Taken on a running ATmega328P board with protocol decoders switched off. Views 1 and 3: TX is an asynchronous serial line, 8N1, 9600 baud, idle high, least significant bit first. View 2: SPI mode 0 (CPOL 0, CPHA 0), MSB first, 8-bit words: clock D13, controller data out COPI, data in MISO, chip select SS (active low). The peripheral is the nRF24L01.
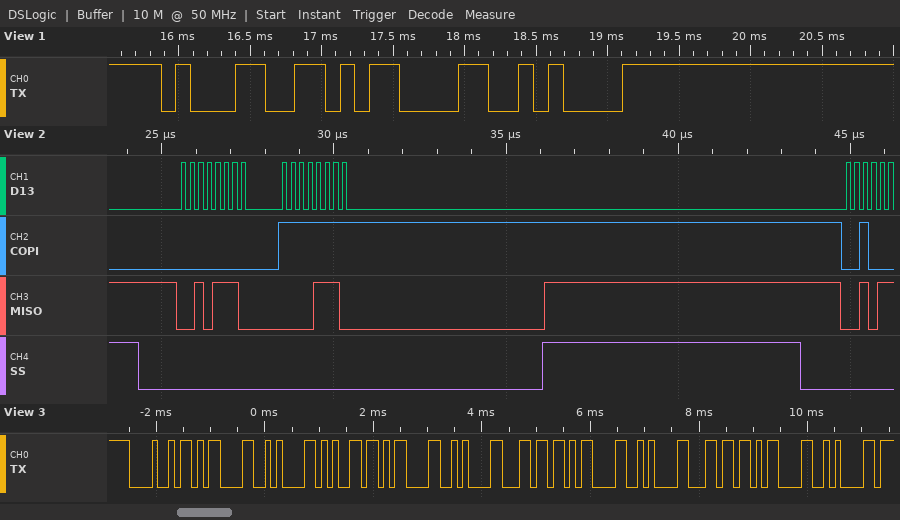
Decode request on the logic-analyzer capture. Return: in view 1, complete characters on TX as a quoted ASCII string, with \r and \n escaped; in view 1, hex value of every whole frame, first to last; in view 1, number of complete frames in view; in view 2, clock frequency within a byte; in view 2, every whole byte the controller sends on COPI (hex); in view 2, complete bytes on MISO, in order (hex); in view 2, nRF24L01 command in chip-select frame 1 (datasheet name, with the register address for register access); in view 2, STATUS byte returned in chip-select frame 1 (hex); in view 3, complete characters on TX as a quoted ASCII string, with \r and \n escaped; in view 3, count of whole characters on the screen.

"1\r\n"
0x31 0x0D 0x0A
3
4 MHz
00 FF
2E 0E
R_REGISTER 0x00
0x2E
"H\r\ne\r\nl\r\nl\r\n"
12
